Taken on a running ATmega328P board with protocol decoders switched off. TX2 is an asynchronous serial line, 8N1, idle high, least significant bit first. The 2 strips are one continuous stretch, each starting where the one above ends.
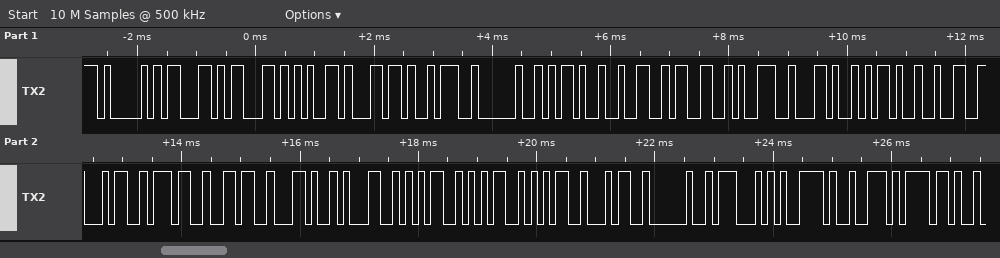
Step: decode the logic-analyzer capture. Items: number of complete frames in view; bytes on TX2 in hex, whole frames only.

28
0x41 0x63 0x63 0x65 0x6C 0x3A 0x20 0x2D 0x32 0x33 0x39 0x2C 0x2D 0x32 0x34 0x37 0x36 0x2C 0x31 0x35 0x35 0x35 0x34 0x20 0x47 0x79 0x72 0x6F
